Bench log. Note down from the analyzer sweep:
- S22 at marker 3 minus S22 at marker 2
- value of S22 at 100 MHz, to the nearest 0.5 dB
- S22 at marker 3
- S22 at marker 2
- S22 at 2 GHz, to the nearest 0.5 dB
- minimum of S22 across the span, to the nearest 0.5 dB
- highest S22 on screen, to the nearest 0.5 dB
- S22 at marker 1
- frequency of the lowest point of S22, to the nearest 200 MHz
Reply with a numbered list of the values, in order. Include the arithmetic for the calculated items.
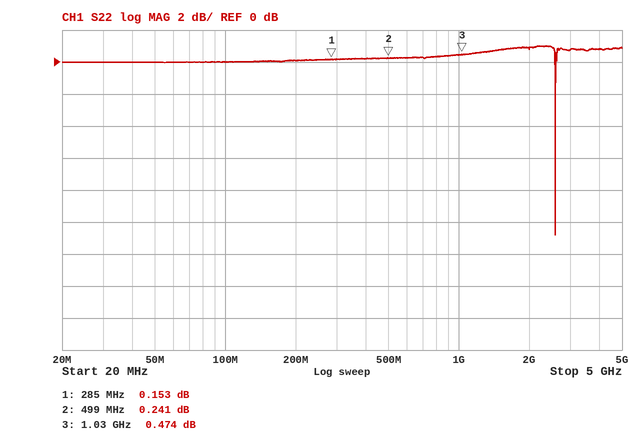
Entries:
1. 0.474 − (0.241) = 0.233 dB
2. 0.0 dB
3. 0.474 dB
4. 0.241 dB
5. 1.0 dB
6. -11.0 dB
7. 1.0 dB
8. 0.153 dB
9. 2.6 GHz
